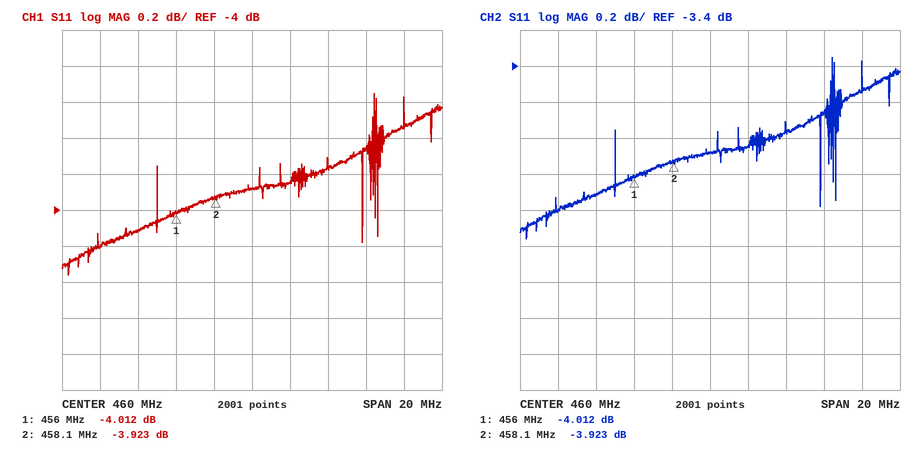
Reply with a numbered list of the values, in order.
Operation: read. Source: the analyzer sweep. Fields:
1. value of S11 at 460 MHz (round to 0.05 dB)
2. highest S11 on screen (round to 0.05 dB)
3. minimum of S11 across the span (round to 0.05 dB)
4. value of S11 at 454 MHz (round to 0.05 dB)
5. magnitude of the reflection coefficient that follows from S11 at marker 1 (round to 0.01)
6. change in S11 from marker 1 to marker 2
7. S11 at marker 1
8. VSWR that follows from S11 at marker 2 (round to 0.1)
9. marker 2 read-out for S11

1. -3.90 dB
2. -3.35 dB
3. -4.35 dB
4. -4.10 dB
5. 0.63
6. 0.089 dB
7. -4.012 dB
8. 4.5
9. -3.923 dB
